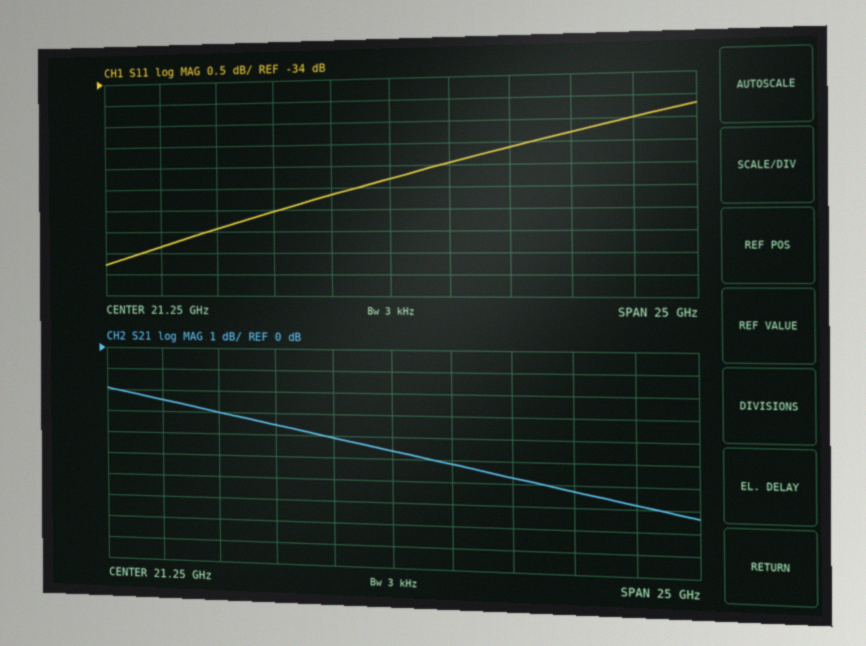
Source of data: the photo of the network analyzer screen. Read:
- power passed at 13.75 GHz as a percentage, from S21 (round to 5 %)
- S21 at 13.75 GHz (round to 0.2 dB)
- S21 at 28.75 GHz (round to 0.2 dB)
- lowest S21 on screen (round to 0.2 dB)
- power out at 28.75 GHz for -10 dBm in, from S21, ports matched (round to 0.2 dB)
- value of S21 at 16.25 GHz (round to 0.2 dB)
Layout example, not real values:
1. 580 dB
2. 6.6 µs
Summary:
1. 50 %
2. -3.0 dB
3. -6.2 dB
4. -7.4 dB
5. -16.2 dBm
6. -3.6 dB
